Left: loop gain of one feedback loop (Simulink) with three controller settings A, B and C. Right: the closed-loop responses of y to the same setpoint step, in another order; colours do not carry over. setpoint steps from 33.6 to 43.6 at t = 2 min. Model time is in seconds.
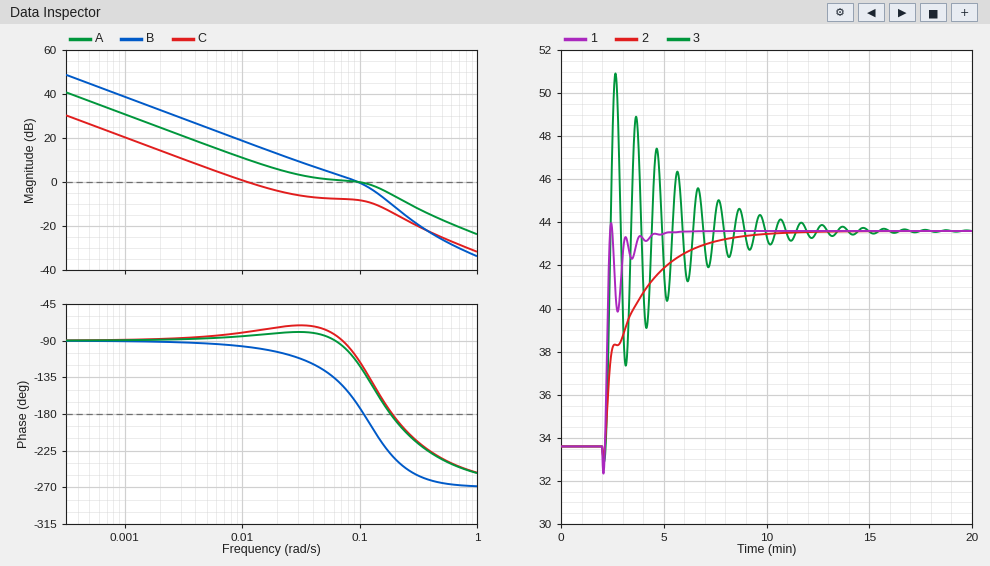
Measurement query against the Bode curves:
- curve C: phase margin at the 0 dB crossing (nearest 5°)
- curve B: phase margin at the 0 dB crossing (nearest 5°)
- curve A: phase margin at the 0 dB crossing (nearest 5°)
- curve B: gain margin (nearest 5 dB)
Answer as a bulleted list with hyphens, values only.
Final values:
- 100°
- 10°
- 60°
- 0 dB
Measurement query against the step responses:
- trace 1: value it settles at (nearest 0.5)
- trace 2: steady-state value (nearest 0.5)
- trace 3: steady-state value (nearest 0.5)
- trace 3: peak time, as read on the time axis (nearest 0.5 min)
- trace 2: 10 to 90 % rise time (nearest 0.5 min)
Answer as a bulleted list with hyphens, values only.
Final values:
- 43.5
- 43.5
- 43.5
- 2.5 min
- 4.0 min
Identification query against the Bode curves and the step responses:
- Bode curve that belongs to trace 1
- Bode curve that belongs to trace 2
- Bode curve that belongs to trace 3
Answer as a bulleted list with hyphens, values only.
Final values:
- A
- C
- B
